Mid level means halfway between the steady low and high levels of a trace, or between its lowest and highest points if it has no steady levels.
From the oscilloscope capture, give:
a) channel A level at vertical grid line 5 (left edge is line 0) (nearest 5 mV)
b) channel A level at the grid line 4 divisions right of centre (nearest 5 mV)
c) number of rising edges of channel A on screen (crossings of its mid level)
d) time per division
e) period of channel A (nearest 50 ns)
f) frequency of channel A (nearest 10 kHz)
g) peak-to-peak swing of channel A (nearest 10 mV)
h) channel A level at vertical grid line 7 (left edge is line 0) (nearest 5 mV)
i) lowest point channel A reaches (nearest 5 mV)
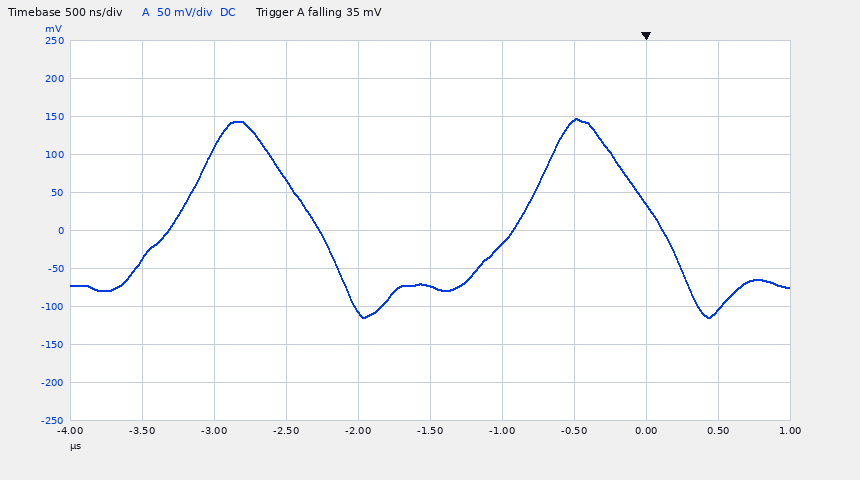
-75 mV
-105 mV
2
500 ns
2.40 µs
420 kHz
260 mV
145 mV
-115 mV
